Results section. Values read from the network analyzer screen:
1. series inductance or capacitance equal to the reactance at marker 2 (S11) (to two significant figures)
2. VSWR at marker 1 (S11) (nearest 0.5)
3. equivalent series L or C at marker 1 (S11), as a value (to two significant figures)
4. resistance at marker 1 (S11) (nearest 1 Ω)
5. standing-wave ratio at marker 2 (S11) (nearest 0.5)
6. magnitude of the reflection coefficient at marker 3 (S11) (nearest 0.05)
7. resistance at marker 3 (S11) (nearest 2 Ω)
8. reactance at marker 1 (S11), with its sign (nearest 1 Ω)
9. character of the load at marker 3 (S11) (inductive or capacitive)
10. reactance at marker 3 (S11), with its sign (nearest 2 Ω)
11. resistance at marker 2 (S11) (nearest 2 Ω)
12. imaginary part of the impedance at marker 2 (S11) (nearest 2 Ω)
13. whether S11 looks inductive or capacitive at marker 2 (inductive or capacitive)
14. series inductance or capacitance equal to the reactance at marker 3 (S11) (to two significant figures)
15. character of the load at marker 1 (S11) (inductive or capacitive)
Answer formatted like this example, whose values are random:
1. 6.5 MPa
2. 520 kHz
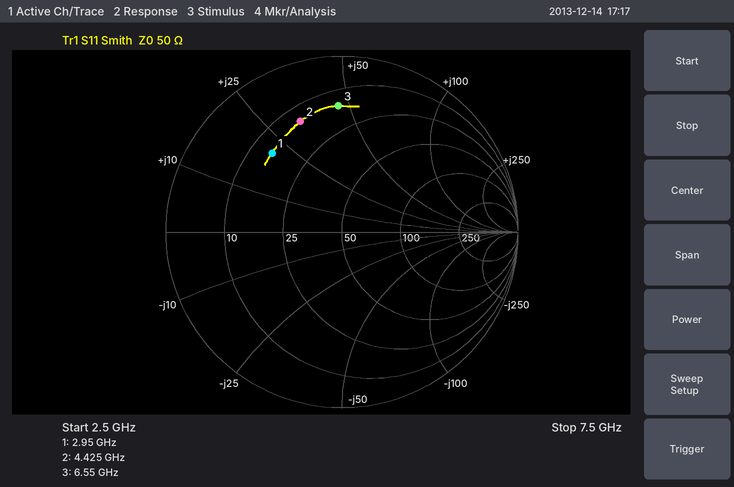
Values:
1. 1.2 nH
2. 4.0
3. 1.1 nH
4. 15 Ω
5. 5.0
6. 0.70
7. 16 Ω
8. +21 Ω
9. inductive
10. +46 Ω
11. 14 Ω
12. +32 Ω
13. inductive
14. 1.1 nH
15. inductive
